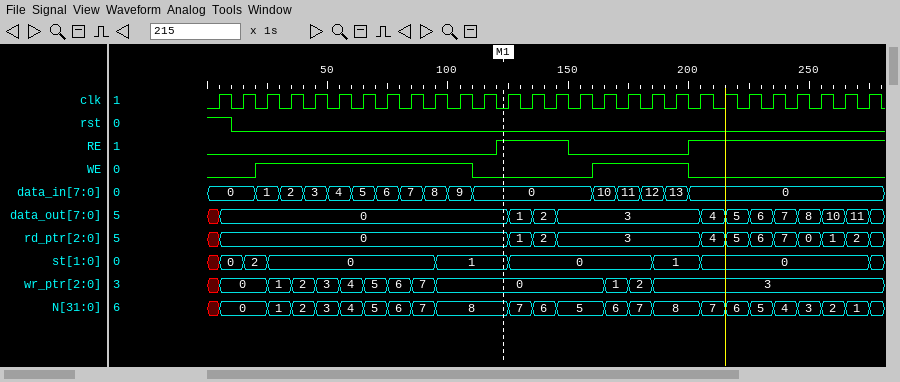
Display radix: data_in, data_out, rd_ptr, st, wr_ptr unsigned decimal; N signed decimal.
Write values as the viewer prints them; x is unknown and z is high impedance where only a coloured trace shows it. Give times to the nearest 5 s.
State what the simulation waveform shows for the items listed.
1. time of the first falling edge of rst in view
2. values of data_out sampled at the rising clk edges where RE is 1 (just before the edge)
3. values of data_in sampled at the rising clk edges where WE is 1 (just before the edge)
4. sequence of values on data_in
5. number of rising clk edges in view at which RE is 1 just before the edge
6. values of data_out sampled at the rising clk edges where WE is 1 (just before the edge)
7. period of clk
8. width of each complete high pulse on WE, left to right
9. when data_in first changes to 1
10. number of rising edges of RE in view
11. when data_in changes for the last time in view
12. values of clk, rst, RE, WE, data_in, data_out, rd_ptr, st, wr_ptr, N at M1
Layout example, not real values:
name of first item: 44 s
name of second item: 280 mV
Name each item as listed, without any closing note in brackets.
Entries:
time of the first falling edge of rst in view: 10 s
values of data_out sampled at the rising clk edges where RE is 1: 0, 1, 2, 3, 4, 5, 6, 7, 8, 10, 11
values of data_in sampled at the rising clk edges where WE is 1: 1, 2, 3, 4, 5, 6, 7, 8, 9, 10, 11, 12, 13
sequence of values on data_in: 0, 1, 2, 3, 4, 5, 6, 7, 8, 9, 0, 10, 11, 12, 13, 0
number of rising clk edges in view at which RE is 1 just before the edge: 11
values of data_out sampled at the rising clk edges where WE is 1: 0, 0, 0, 0, 0, 0, 0, 0, 0, 3, 3, 3, 3
period of clk: 10 s
width of each complete high pulse on WE, left to right: 90 s, 40 s
when data_in first changes to 1: 20 s
number of rising edges of RE in view: 2
when data_in changes for the last time in view: 200 s
values of clk, rst, RE, WE, data_in, data_out, rd_ptr, st, wr_ptr, N at M1: clk=0, rst=0, RE=1, WE=0, data_in=0, data_out=0, rd_ptr=0, st=1, wr_ptr=0, N=8
